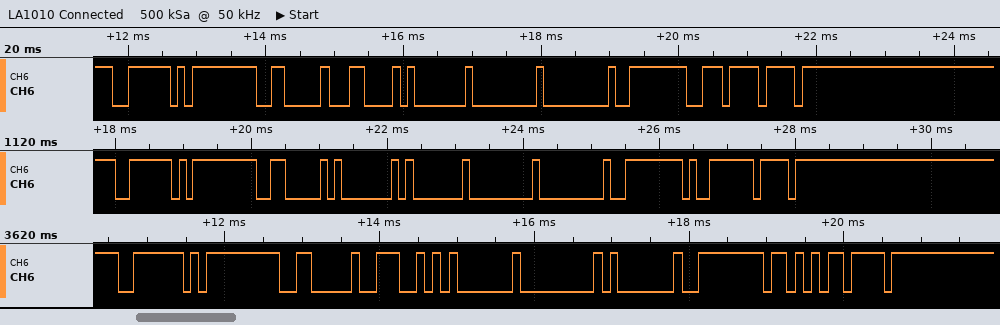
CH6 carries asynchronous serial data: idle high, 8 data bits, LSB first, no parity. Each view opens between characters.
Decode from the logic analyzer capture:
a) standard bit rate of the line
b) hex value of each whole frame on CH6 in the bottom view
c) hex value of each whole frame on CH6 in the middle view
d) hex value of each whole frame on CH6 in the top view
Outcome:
9600 baud
7E, FF, 06, 4E, 01, 00, 01, FE, AB, EF
7E, FF, 06, 01, 01, 00, 00, FE, F9, EF
7E, FF, 06, 0C, 01, 00, 00, FE, EE, EF
